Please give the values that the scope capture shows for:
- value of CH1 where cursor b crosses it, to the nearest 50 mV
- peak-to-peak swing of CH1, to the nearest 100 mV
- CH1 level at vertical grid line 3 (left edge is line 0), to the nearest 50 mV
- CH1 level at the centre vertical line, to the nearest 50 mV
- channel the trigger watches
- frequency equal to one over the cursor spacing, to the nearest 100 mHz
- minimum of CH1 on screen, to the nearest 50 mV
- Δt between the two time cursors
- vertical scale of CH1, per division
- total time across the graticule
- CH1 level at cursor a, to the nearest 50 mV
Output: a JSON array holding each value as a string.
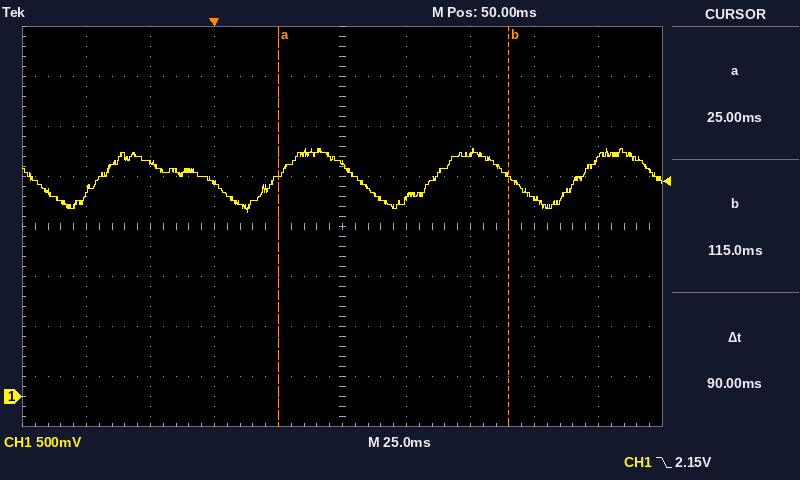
["2.20 V", "600 mV", "2.15 V", "2.30 V", "CH1", "11.1 Hz", "1.85 V", "90 ms", "500 mV", "250 ms", "2.20 V"]
